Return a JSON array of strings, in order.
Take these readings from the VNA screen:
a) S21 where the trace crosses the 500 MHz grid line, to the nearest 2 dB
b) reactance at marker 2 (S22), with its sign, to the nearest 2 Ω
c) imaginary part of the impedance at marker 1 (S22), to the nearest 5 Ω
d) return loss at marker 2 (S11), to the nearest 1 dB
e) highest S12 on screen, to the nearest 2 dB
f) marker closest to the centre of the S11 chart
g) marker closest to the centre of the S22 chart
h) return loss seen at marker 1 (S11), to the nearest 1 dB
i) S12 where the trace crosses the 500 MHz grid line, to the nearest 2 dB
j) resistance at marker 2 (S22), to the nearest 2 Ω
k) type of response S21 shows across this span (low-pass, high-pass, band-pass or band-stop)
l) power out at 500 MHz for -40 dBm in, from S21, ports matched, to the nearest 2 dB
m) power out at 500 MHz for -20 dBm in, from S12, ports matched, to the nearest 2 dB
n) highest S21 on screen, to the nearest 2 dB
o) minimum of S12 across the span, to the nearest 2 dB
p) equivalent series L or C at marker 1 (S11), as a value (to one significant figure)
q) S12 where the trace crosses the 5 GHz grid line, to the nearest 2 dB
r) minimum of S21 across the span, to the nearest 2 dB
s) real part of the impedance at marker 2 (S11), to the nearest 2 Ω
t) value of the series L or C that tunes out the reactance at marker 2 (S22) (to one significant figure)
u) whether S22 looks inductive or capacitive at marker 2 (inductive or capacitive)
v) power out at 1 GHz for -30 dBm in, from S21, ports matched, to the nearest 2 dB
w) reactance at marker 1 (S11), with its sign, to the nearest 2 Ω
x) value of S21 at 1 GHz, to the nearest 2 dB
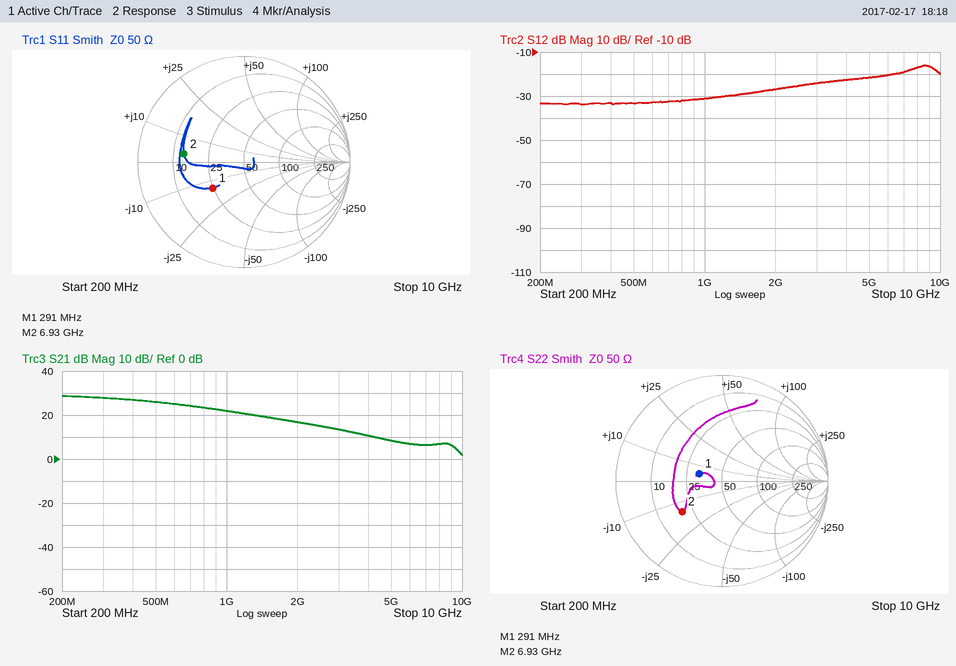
["26 dB", "-14 Ω", "+5 Ω", "5 dB", "-16 dB", "marker 1", "marker 1", "8 dB", "-34 dB", "20 Ω", "low-pass", "-14 dBm", "-54 dBm", "28 dB", "-34 dB", "40 pF", "-22 dB", "2 dB", "14 Ω", "300 pH", "capacitive", "-8 dBm", "-14 Ω", "22 dB"]
